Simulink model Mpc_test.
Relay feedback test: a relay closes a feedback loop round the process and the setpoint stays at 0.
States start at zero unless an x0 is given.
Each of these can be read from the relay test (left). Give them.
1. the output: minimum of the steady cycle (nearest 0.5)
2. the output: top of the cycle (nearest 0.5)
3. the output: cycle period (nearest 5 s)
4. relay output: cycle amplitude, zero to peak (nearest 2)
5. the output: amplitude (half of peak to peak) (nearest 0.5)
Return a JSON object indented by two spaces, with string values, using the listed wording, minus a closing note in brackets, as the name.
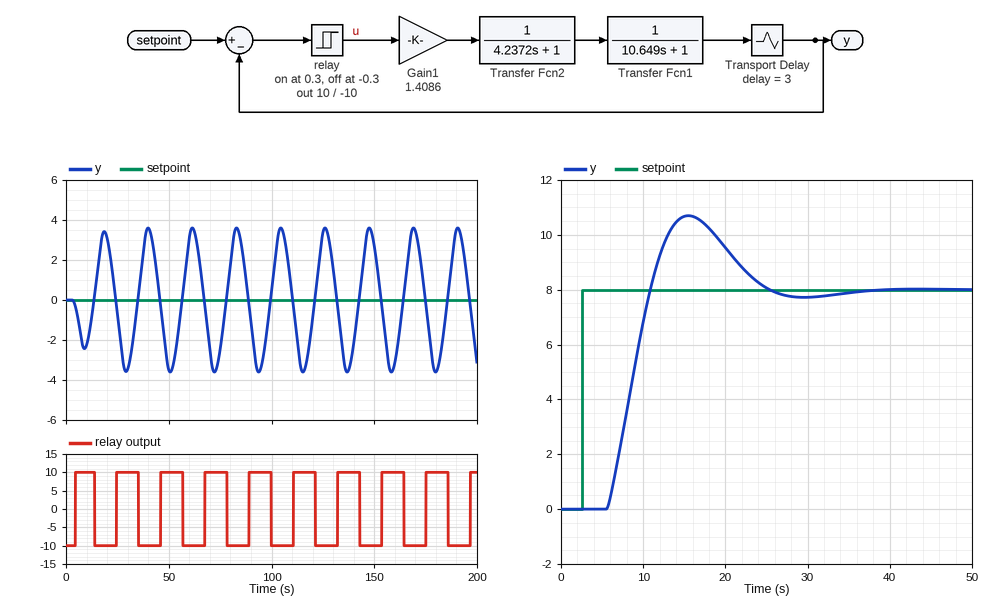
{
  "the output: minimum of the steady cycle": "-3.5",
  "the output: top of the cycle": "3.5",
  "the output: cycle period": "20 s",
  "relay output: cycle amplitude, zero to peak": "10",
  "the output: amplitude (half of peak to peak)": "3.5"
}
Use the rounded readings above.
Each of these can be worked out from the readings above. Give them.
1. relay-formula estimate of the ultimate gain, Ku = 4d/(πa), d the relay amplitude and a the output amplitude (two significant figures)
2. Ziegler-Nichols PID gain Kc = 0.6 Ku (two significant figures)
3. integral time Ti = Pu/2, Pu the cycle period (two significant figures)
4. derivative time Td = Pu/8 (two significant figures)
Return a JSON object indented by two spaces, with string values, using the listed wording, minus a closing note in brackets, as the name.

{
  "relay-formula estimate of the ultimate gain, Ku = 4d/(πa), d the relay amplitude and a the output amplitude": "3.6",
  "Ziegler-Nichols PID gain Kc = 0.6 Ku": "2.2",
  "integral time Ti = Pu/2, Pu the cycle period": "10 s",
  "derivative time Td = Pu/8": "2.5 s"
}
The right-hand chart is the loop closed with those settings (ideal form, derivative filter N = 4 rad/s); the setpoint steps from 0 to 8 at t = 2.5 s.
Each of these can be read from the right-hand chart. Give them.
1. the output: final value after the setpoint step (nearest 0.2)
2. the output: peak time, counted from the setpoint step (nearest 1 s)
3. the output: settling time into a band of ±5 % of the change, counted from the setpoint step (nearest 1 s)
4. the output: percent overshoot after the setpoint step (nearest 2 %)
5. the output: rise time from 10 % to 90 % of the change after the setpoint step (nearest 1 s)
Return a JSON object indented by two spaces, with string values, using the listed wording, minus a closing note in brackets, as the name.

{
  "the output: final value after the setpoint step": "8.0",
  "the output: peak time, counted from the setpoint step": "13 s",
  "the output: settling time into a band of ±5 % of the change, counted from the setpoint step": "21 s",
  "the output: percent overshoot after the setpoint step": "34 %",
  "the output: rise time from 10 % to 90 % of the change after the setpoint step": "4 s"
}
